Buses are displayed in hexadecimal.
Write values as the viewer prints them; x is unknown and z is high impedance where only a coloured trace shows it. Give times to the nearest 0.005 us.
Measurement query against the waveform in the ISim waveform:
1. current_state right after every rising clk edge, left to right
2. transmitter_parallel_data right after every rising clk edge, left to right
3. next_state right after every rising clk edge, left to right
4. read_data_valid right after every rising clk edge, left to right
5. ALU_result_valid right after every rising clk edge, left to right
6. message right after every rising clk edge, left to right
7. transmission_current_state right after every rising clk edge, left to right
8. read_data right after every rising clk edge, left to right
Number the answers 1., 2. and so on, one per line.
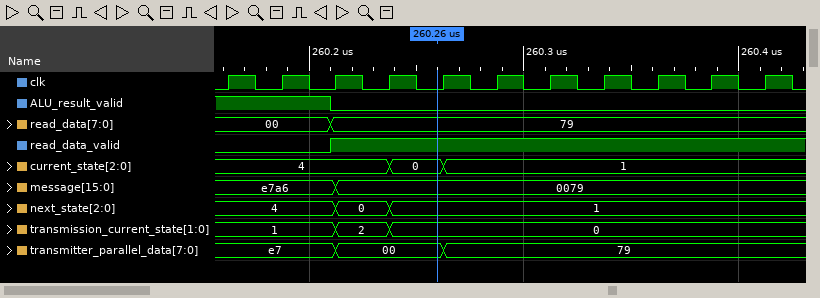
1. 4, 4, 4, 0, 1, 1, 1, 1, 1, 1, 1
2. e7, e7, 00, 00, 79, 79, 79, 79, 79, 79, 79
3. 4, 4, 0, 1, 1, 1, 1, 1, 1, 1, 1
4. 0 0 1 1 1 1 1 1 1 1 1
5. 1 1 0 0 0 0 0 0 0 0 0
6. e7a6, e7a6, 0079, 0079, 0079, 0079, 0079, 0079, 0079, 0079, 0079
7. 1, 1, 2, 0, 0, 0, 0, 0, 0, 0, 0
8. 00, 00, 79, 79, 79, 79, 79, 79, 79, 79, 79
